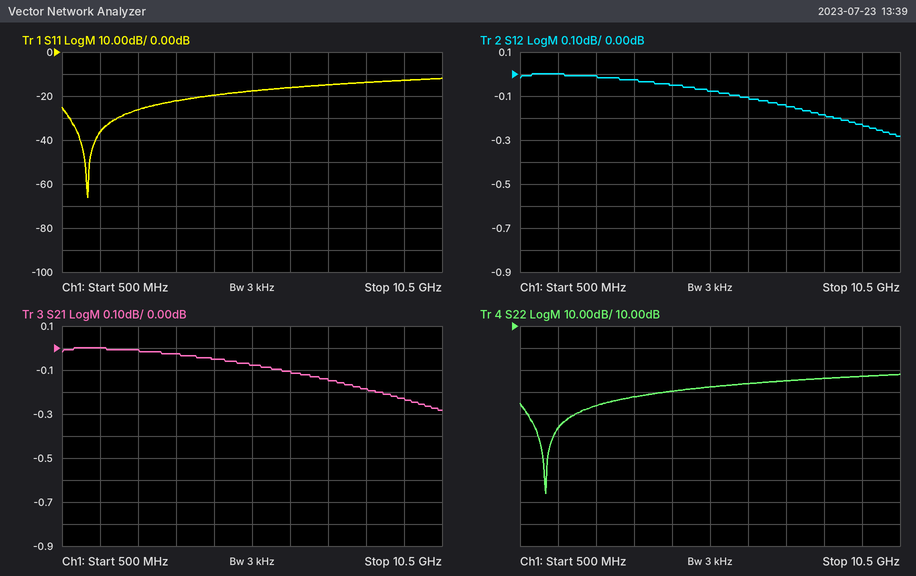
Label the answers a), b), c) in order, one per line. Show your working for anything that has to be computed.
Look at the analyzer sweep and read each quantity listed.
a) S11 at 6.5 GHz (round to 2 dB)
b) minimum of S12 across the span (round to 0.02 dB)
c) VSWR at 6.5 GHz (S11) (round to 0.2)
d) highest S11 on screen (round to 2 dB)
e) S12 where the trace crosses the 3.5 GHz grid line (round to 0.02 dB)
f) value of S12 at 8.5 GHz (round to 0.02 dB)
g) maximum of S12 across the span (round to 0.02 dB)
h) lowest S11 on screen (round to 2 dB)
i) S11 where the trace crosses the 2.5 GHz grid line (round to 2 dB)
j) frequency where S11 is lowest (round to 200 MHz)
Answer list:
a) -16 dB
b) -0.28 dB
c) |Γ| = 10^(-16/20) = 0.1585; VSWR = (1 + 0.1585)/(1 − 0.1585) ≈ 1.4
d) -12 dB
e) -0.02 dB
f) -0.18 dB
g) 0.00 dB
h) -66 dB
i) -26 dB
j) 1.2 GHz
